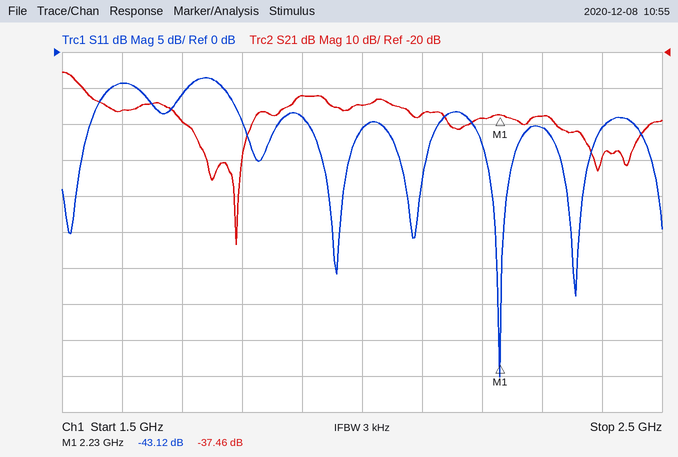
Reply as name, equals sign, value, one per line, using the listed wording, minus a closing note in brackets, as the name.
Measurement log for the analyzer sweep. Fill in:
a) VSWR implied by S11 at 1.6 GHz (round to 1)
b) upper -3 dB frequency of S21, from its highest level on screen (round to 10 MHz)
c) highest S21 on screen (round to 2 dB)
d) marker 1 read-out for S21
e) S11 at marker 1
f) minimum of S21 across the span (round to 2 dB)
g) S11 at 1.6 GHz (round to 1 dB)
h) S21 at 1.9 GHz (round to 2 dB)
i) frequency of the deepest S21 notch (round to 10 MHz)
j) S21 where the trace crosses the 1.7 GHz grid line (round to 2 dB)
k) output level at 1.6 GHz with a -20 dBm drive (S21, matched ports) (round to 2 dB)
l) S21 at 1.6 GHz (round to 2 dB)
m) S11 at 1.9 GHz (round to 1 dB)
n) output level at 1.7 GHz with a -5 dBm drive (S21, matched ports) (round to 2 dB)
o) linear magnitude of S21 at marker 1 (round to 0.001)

VSWR implied by S11 at 1.6 GHz = 4
upper -3 dB frequency of S21, from its highest level on screen = 1.53 GHz
highest S21 on screen = -26 dB
marker 1 read-out for S21 = -37.46 dB
S11 at marker 1 = -43.12 dB
minimum of S21 across the span = -74 dB
S11 at 1.6 GHz = -4 dB
S21 at 1.9 GHz = -32 dB
frequency of the deepest S21 notch = 1.79 GHz
S21 where the trace crosses the 1.7 GHz grid line = -40 dB
output level at 1.6 GHz with a -20 dBm drive (S21, matched ports) = -56 dBm
S21 at 1.6 GHz = -36 dB
S11 at 1.9 GHz = -9 dB
output level at 1.7 GHz with a -5 dBm drive (S21, matched ports) = -44 dBm
linear magnitude of S21 at marker 1 = 0.013
